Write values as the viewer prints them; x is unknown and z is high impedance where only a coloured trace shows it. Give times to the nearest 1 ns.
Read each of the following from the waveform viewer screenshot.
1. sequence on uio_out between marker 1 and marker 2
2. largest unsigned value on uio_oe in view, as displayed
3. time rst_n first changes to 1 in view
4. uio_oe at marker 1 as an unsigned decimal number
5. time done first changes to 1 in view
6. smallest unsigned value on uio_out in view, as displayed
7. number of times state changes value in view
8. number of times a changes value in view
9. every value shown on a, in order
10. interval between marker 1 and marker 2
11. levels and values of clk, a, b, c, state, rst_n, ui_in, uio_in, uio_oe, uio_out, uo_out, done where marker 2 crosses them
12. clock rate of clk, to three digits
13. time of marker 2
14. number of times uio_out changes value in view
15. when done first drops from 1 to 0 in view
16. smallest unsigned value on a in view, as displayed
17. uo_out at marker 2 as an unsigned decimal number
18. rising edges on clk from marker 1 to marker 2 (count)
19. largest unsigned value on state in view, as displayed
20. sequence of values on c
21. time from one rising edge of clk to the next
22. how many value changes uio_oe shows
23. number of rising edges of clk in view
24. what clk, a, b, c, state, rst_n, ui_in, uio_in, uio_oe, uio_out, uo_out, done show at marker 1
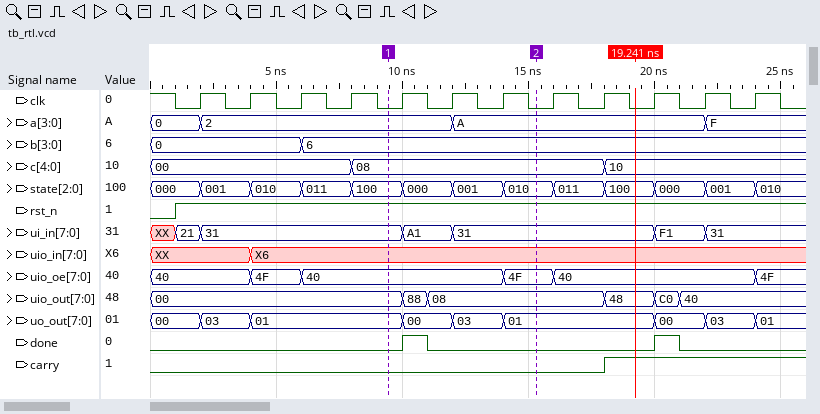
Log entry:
00, 88, 08
4F
1 ns
64
10 ns
00
12
3
0, 2, A, F
6 ns
clk=0, a=A, b=6, c=08, state=010, rst_n=1, ui_in=31, uio_in=X6, uio_oe=4F, uio_out=08, uo_out=01, done=0
500 MHz
15 ns
5
11 ns
0
1
3
100
00, 08, 10
2 ns
5
12
clk=0, a=2, b=6, c=08, state=100, rst_n=1, ui_in=31, uio_in=X6, uio_oe=40, uio_out=00, uo_out=01, done=0
